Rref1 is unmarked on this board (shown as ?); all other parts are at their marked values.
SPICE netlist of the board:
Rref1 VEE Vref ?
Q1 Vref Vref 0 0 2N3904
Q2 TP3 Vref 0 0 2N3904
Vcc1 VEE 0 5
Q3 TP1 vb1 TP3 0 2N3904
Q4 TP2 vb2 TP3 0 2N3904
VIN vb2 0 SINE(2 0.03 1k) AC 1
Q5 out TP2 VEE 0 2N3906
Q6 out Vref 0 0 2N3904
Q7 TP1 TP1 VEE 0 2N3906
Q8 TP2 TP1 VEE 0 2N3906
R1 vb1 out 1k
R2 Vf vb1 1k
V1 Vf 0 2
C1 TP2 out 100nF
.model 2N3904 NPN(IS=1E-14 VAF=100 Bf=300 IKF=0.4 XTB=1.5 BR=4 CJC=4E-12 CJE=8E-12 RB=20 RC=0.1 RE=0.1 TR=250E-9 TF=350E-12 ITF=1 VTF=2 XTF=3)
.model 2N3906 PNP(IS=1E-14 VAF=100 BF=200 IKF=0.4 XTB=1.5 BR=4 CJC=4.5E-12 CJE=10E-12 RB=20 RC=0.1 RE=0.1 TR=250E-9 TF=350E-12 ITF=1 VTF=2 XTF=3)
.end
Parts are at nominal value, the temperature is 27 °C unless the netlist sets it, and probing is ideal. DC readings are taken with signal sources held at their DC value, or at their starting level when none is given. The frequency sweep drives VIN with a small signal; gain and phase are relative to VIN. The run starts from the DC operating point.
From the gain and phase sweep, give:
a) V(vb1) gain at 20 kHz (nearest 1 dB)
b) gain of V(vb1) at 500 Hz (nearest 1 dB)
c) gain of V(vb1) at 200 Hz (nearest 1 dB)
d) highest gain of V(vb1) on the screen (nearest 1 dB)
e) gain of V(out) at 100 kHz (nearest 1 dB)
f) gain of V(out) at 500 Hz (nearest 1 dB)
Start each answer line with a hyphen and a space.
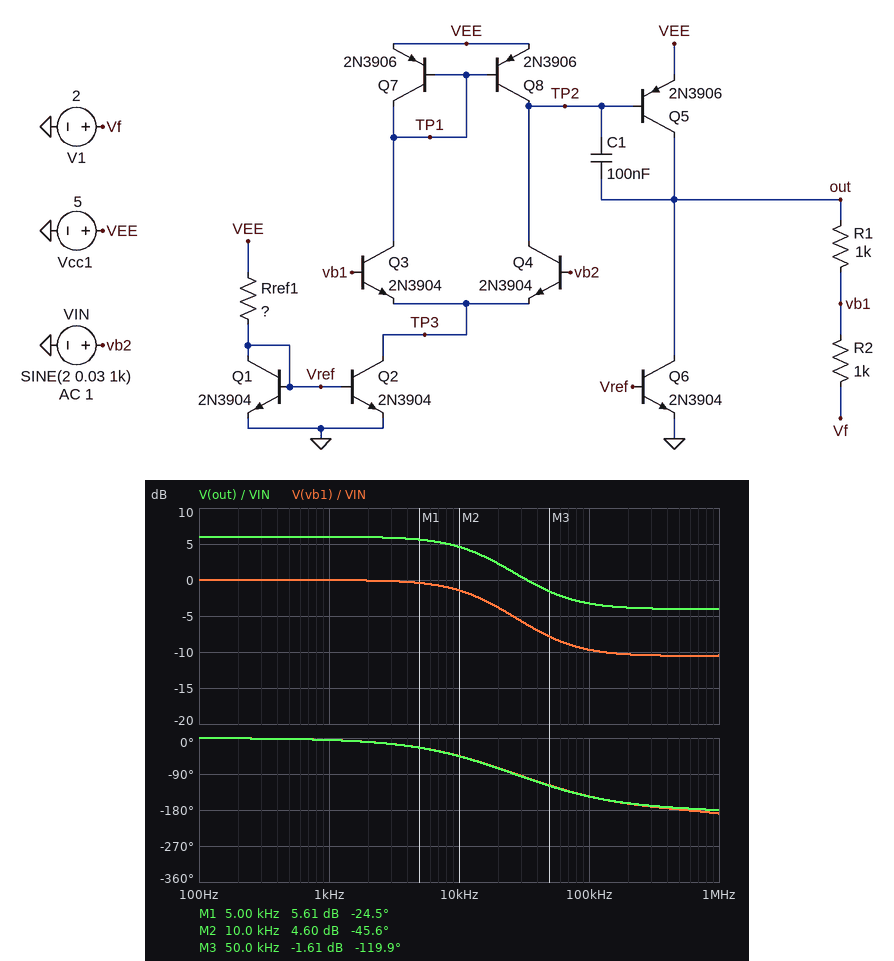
- -4 dB
- 0 dB
- 0 dB
- 0 dB
- -3 dB
- 6 dB
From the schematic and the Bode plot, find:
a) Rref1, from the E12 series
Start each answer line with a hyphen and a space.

- 5.6 kΩ
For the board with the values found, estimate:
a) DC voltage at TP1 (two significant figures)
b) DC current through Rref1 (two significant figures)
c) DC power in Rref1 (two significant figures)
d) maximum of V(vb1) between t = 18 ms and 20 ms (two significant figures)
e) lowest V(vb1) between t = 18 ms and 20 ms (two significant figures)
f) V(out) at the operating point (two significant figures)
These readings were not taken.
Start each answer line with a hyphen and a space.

- 4.4 V
- 780 µA
- 3.4 mW
- 2.0 V
- 2.0 V
- 2.0 V
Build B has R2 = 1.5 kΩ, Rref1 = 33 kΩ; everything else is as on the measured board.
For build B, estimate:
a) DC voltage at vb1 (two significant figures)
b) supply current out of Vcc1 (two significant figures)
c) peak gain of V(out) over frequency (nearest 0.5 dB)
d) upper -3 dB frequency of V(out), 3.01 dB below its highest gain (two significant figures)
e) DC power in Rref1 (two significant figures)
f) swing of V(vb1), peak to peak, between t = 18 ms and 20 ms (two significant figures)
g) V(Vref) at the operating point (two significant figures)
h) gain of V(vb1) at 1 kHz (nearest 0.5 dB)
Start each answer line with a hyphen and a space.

- 2.0 V
- 400 µA
- 4.5 dB
- 3.6 kHz
- 590 µW
- 57 mV
- 600 mV
- -0.5 dB
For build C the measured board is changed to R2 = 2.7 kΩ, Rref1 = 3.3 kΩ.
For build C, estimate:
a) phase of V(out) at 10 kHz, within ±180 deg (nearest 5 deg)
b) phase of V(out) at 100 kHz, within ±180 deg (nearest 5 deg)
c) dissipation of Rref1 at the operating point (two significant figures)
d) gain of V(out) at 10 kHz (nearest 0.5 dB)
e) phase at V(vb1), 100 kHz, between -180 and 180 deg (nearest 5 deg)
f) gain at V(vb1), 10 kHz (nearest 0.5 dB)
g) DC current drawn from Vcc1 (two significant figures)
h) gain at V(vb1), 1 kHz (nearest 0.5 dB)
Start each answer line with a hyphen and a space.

- -20 deg
- -120 deg
- 5.7 mW
- 2.5 dB
- -115 deg
- 0 dB
- 3.9 mA
- 0 dB
